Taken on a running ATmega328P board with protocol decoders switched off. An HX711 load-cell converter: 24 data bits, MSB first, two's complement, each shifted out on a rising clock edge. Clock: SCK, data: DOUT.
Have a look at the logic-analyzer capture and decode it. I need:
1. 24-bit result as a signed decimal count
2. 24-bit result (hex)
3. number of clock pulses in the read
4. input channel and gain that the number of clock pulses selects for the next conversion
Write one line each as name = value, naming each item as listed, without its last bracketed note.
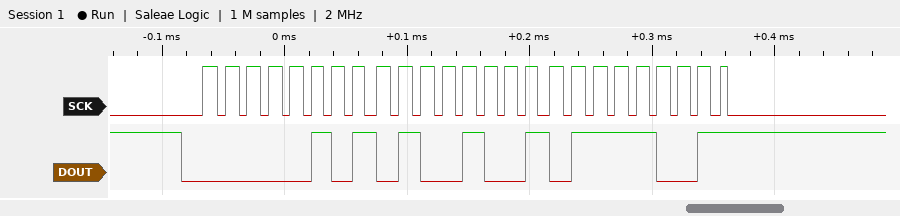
24-bit result as a signed decimal count = 346489
24-bit result = 0x054979
number of clock pulses in the read = 25
input channel and gain that the number of clock pulses selects for the next conversion = channel A, gain 128
